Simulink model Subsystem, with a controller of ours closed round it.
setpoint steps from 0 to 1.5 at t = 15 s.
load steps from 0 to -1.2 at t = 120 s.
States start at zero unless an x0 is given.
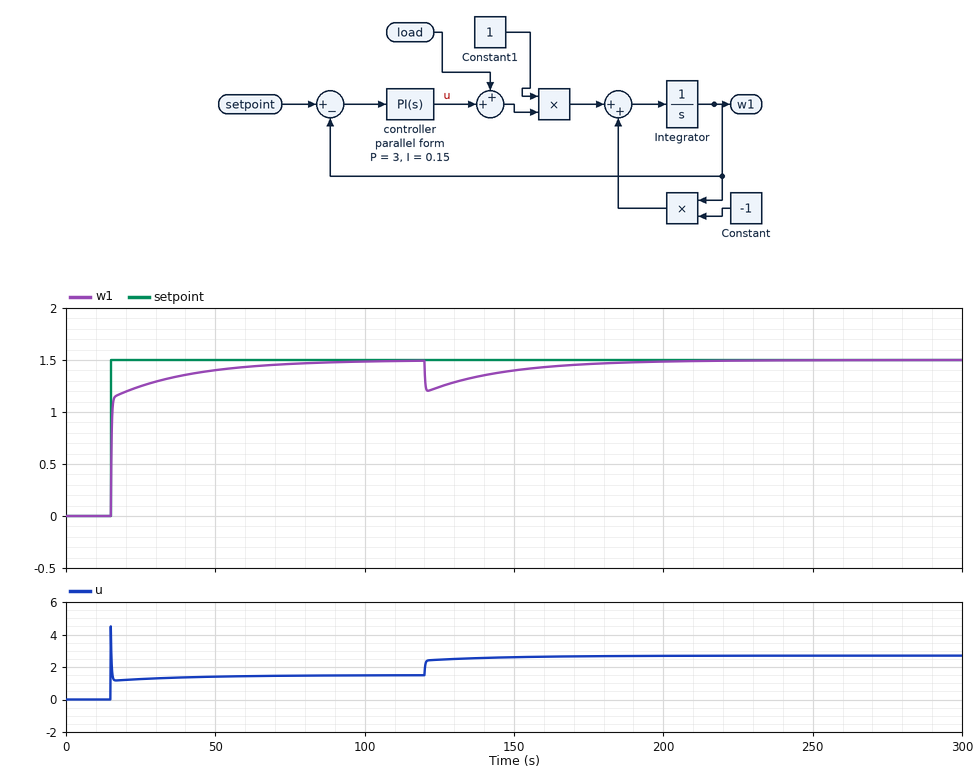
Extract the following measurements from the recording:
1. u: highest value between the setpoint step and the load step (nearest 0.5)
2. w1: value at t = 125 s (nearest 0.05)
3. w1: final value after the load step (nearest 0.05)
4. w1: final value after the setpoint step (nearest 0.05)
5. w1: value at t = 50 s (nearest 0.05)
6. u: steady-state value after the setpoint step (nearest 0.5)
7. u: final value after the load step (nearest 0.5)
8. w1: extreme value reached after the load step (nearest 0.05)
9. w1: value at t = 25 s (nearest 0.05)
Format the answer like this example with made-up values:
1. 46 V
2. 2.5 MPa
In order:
1. 4.5
2. 1.25
3. 1.50
4. 1.50
5. 1.40
6. 1.5
7. 2.5
8. 1.20
9. 1.25
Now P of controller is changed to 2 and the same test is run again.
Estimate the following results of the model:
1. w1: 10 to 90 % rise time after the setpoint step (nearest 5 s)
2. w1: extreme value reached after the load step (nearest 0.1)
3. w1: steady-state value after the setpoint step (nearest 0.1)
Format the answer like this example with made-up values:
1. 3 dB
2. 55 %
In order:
1. 25 s
2. 1.1
3. 1.5
